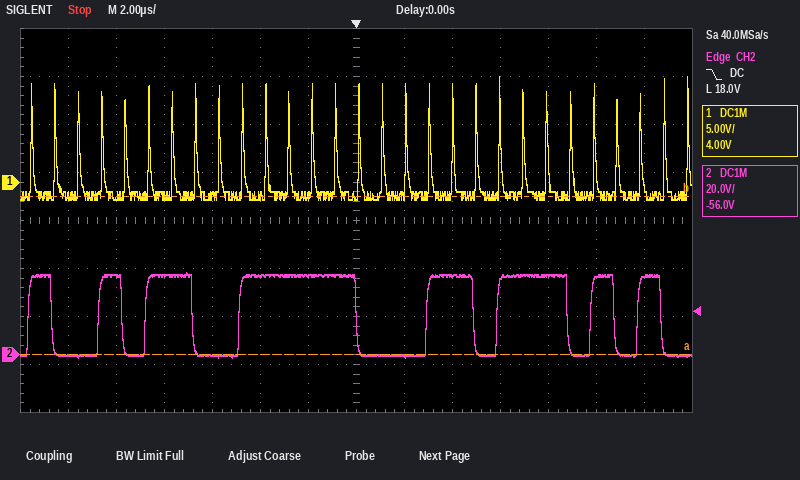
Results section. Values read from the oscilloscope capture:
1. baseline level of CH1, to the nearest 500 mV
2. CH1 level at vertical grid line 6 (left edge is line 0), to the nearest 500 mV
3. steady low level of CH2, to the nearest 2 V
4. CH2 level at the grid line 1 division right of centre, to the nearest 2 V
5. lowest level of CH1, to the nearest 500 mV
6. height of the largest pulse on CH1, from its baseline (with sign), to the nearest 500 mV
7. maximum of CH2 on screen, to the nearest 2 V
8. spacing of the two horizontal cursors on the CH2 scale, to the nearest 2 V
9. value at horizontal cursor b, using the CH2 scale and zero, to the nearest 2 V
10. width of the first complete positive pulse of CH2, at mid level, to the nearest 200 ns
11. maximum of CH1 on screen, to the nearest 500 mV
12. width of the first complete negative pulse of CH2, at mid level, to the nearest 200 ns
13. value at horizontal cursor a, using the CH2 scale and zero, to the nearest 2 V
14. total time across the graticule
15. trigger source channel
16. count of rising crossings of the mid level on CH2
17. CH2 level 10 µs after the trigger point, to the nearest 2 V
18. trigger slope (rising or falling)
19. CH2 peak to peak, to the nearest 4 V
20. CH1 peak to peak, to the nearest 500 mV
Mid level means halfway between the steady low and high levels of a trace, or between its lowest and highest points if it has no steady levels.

-1.5 V
-1.5 V
0 V
0 V
-2.0 V
+12.5 V
34 V
66 V
66 V
1.0 µs
11.0 V
2.0 µs
0 V
28 µs
CH2
8
32 V
falling
36 V
13.0 V
